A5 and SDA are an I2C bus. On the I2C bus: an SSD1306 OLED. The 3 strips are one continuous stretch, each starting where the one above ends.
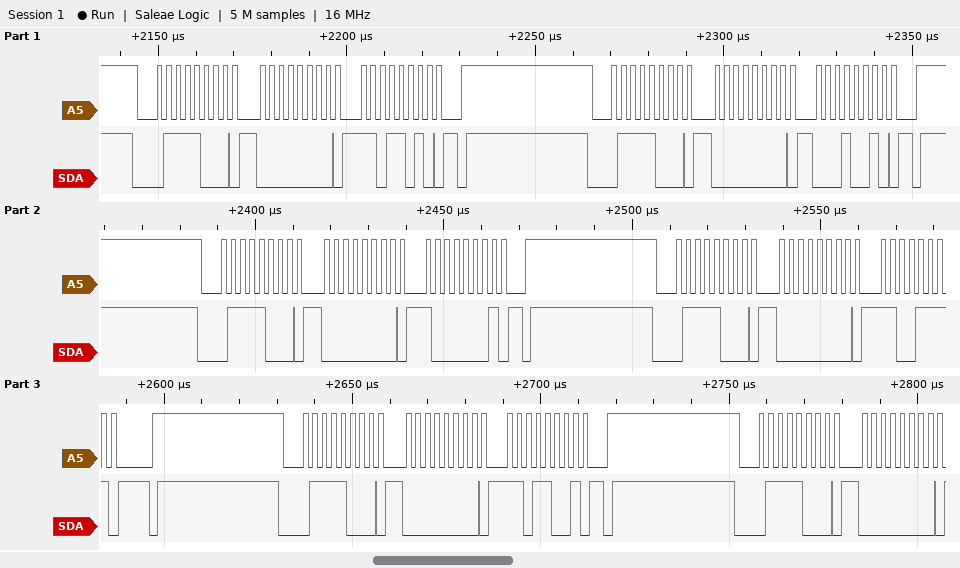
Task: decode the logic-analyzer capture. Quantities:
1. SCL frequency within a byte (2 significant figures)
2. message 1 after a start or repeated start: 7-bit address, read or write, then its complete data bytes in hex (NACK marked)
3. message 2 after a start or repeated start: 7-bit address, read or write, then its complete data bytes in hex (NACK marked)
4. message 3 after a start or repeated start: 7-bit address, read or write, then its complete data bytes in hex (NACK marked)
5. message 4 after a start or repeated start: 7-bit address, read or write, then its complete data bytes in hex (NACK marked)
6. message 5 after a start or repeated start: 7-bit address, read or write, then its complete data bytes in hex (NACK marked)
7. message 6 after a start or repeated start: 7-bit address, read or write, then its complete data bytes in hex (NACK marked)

400 kHz
0x3C write: 00 DA
0x3C write: 00 12
0x3C write: 00 81
0x3C write: 00 CF
0x3C write: 00 D9
0x3C write: 00
